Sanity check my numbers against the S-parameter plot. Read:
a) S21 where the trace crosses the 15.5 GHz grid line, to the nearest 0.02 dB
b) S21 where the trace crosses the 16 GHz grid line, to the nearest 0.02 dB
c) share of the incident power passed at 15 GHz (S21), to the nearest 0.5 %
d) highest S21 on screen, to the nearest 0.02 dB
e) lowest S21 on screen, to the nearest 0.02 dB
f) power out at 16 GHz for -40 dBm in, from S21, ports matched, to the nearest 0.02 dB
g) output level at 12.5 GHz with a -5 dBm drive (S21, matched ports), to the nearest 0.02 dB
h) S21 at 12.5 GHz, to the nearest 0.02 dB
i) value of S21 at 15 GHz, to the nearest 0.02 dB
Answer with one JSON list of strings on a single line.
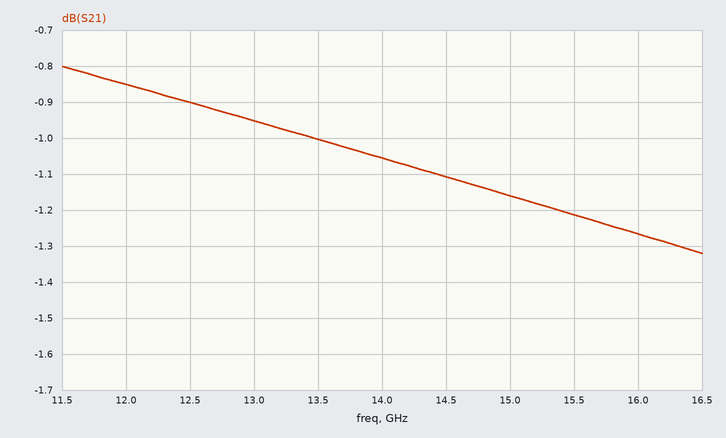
["-1.22 dB", "-1.26 dB", "76.5 %", "-0.80 dB", "-1.32 dB", "-41.26 dBm", "-5.90 dBm", "-0.90 dB", "-1.16 dB"]
